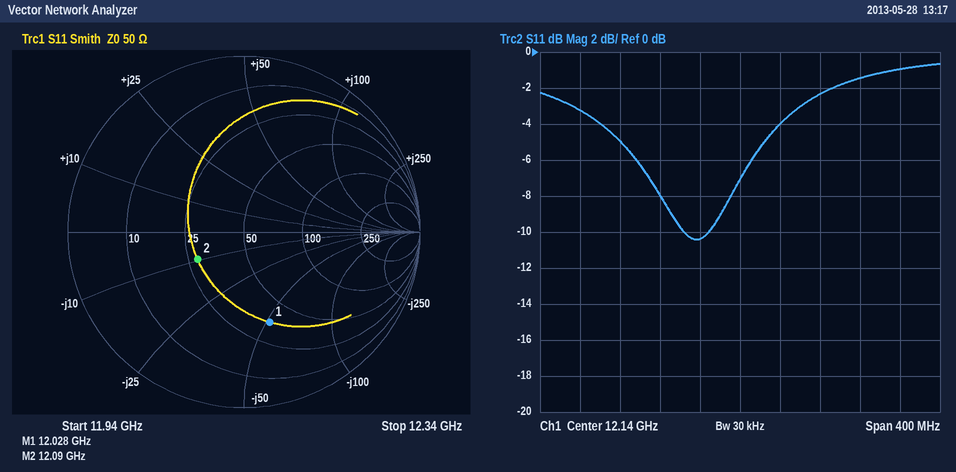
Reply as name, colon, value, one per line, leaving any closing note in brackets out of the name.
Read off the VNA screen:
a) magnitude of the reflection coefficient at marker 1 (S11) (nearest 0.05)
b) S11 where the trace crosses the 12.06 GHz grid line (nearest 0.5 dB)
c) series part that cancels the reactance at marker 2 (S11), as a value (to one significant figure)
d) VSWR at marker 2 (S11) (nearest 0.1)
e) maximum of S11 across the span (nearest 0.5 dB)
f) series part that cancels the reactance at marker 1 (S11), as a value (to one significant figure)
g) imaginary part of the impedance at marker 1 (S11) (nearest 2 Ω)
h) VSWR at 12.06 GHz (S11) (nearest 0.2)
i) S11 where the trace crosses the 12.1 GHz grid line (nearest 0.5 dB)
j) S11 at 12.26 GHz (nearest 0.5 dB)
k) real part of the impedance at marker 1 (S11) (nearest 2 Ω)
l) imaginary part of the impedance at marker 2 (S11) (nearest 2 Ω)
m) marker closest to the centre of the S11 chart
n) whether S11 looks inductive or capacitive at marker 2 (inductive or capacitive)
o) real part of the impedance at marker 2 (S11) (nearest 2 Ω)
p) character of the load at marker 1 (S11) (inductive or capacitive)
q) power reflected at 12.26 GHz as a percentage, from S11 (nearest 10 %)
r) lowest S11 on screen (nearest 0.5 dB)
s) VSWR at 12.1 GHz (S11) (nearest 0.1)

magnitude of the reflection coefficient at marker 1 (S11): 0.55
S11 where the trace crosses the 12.06 GHz grid line: -8.0 dB
series part that cancels the reactance at marker 2 (S11), as a value: 100 pH
VSWR at marker 2 (S11): 1.9
maximum of S11 across the span: -0.5 dB
series part that cancels the reactance at marker 1 (S11), as a value: 700 pH
imaginary part of the impedance at marker 1 (S11): -52 Ω
VSWR at 12.06 GHz (S11): 2.4
S11 where the trace crosses the 12.1 GHz grid line: -10.5 dB
S11 at 12.26 GHz: -1.5 dB
real part of the impedance at marker 1 (S11): 36 Ω
imaginary part of the impedance at marker 2 (S11): -10 Ω
marker closest to the centre of the S11 chart: marker 2
whether S11 looks inductive or capacitive at marker 2: capacitive
real part of the impedance at marker 2 (S11): 28 Ω
character of the load at marker 1 (S11): capacitive
power reflected at 12.26 GHz as a percentage, from S11: 70 %
lowest S11 on screen: -10.5 dB
VSWR at 12.1 GHz (S11): 1.9
